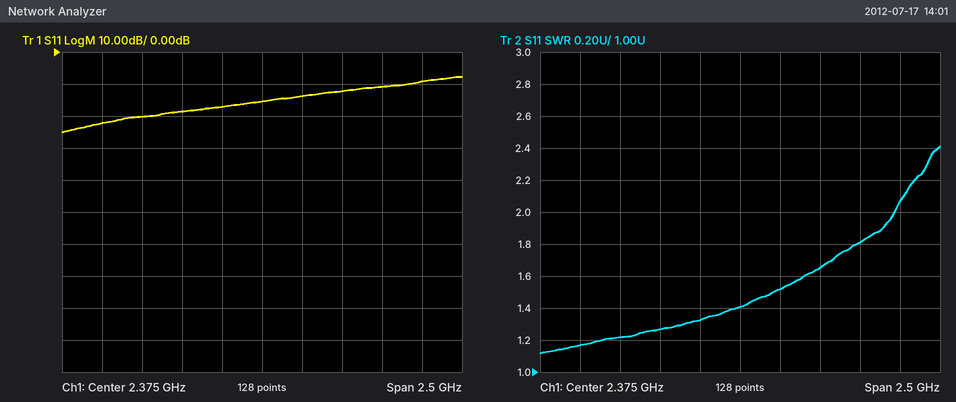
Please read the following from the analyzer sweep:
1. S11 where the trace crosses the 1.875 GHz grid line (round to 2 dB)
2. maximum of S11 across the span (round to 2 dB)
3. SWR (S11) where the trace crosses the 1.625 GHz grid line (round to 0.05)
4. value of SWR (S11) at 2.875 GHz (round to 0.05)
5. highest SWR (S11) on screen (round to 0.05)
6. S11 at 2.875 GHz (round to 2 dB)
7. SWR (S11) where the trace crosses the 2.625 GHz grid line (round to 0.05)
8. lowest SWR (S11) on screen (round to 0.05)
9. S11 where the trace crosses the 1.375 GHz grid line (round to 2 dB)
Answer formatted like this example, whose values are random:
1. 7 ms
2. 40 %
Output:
1. -18 dB
2. -8 dB
3. 1.20
4. 1.65
5. 2.40
6. -12 dB
7. 1.50
8. 1.10
9. -22 dB
